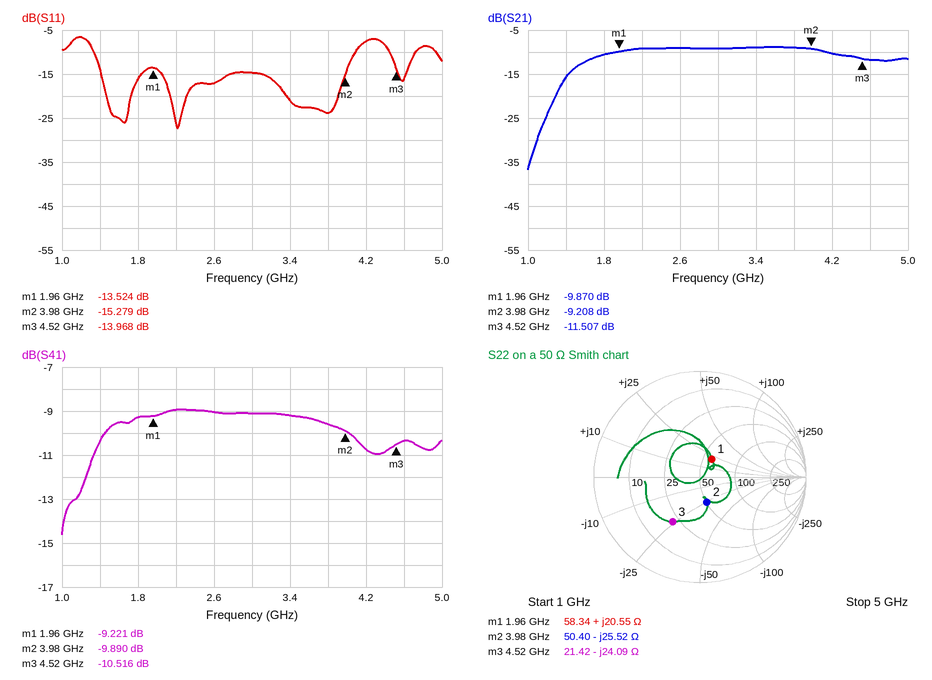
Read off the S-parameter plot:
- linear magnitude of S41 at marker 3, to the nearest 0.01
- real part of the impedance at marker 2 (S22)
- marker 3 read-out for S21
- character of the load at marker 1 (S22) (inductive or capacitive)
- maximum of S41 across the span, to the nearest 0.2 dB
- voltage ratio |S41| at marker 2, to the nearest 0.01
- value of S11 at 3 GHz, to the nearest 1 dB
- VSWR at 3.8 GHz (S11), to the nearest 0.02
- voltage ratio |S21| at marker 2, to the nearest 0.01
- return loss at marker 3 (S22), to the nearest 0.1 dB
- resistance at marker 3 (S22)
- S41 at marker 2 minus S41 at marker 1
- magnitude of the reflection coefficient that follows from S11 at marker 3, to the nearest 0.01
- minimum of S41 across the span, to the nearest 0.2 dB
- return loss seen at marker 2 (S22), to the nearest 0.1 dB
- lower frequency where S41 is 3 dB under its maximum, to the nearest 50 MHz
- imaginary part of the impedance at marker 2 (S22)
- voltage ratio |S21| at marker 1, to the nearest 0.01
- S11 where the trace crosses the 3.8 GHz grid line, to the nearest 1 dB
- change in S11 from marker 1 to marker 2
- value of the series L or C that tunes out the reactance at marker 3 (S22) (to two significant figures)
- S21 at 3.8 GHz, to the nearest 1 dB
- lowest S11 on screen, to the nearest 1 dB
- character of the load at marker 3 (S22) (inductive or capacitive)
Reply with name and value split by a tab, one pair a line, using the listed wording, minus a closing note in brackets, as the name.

linear magnitude of S41 at marker 3, to the nearest 0.01	0.30
real part of the impedance at marker 2	50.40 Ω
marker 3 read-out for S21	-11.507 dB
character of the load at marker 1 (S22)	inductive
maximum of S41 across the span, to the nearest 0.2 dB	-9.0 dB
voltage ratio |S41| at marker 2, to the nearest 0.01	0.32
value of S11 at 3 GHz, to the nearest 1 dB	-15 dB
VSWR at 3.8 GHz (S11), to the nearest 0.02	1.14
voltage ratio |S21| at marker 2, to the nearest 0.01	0.35
return loss at marker 3 (S22), to the nearest 0.1 dB	6.1 dB
resistance at marker 3	21.42 Ω
S41 at marker 2 minus S41 at marker 1	-0.669 dB
magnitude of the reflection coefficient that follows from S11 at marker 3, to the nearest 0.01	0.20
minimum of S41 across the span, to the nearest 0.2 dB	-14.6 dB
return loss seen at marker 2 (S22), to the nearest 0.1 dB	12.2 dB
lower frequency where S41 is 3 dB under its maximum, to the nearest 50 MHz	1.25 GHz
imaginary part of the impedance at marker 2	-25.52 Ω
voltage ratio |S21| at marker 1, to the nearest 0.01	0.32
S11 where the trace crosses the 3.8 GHz grid line, to the nearest 1 dB	-24 dB
change in S11 from marker 1 to marker 2	-1.755 dB
value of the series L or C that tunes out the reactance at marker 3 (S22)	850 pH
S21 at 3.8 GHz, to the nearest 1 dB	-9 dB
lowest S11 on screen, to the nearest 1 dB	-27 dB
character of the load at marker 3 (S22)	capacitive
